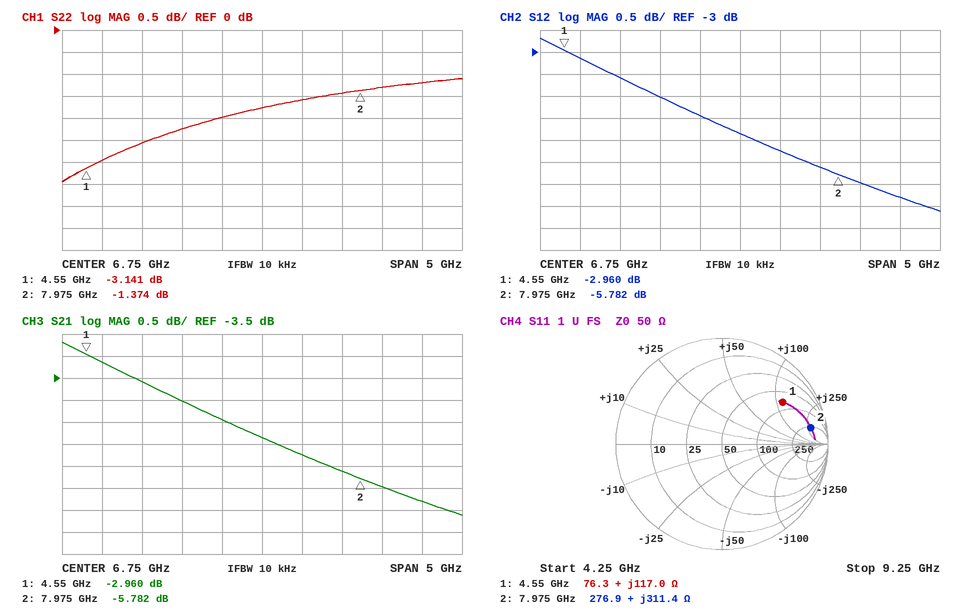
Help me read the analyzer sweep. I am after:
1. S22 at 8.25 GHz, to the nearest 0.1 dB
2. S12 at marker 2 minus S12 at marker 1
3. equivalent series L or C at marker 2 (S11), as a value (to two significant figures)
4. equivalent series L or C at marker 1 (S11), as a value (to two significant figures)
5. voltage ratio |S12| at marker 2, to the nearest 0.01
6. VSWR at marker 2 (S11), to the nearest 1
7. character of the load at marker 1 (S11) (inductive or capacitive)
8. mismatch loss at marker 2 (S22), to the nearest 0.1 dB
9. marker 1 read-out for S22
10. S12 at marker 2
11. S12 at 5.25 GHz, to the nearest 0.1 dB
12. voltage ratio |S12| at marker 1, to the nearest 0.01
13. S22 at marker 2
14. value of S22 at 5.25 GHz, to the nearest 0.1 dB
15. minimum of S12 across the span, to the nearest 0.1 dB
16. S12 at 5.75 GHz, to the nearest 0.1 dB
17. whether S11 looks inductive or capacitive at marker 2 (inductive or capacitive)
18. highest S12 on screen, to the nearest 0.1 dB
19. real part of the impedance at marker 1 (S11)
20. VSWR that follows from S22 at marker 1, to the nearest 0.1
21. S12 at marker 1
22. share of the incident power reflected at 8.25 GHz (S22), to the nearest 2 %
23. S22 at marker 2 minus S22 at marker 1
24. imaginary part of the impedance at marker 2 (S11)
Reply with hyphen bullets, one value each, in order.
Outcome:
- -1.3 dB
- -2.822 dB
- 6.2 nH
- 4.1 nH
- 0.51
- 13
- inductive
- 5.7 dB
- -3.141 dB
- -5.782 dB
- -3.6 dB
- 0.71
- -1.374 dB
- -2.6 dB
- -6.6 dB
- -4.0 dB
- inductive
- -2.7 dB
- 76.3 Ω
- 5.6
- -2.960 dB
- 74 %
- 1.767 dB
- +311.4 Ω
